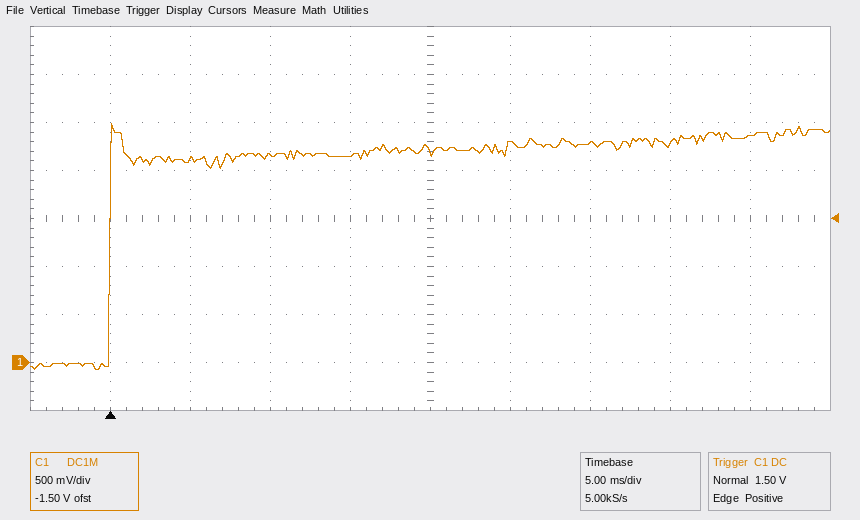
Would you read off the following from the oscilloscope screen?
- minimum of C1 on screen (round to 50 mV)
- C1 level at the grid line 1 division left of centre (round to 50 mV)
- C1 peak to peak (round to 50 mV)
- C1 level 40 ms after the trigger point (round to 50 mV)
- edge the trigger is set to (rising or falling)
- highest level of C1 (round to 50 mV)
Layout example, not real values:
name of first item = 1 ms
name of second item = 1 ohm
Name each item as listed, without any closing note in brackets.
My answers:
minimum of C1 on screen = -50 mV
C1 level at the grid line 1 division left of centre = 2.15 V
C1 peak to peak = 2.55 V
C1 level 40 ms after the trigger point = 2.35 V
edge the trigger is set to = rising
highest level of C1 = 2.50 V
